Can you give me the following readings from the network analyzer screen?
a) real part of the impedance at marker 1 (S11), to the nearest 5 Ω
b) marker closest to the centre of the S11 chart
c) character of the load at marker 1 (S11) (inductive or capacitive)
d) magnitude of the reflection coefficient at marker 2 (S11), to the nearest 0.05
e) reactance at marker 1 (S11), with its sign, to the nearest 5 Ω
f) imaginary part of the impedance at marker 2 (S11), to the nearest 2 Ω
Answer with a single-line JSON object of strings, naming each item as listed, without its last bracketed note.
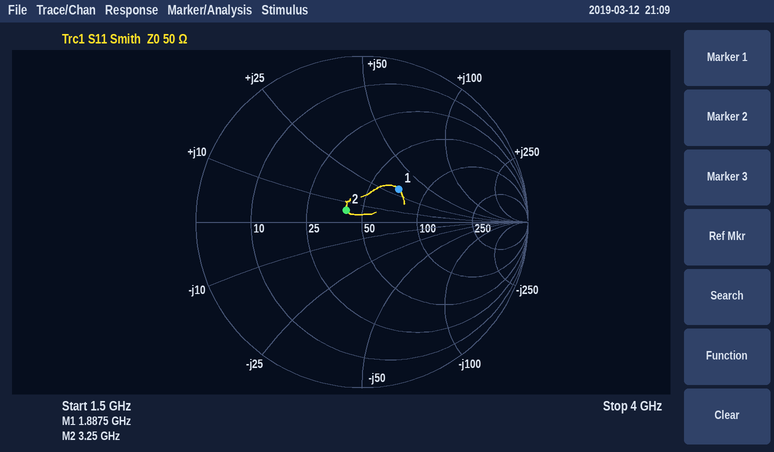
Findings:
{"real part of the impedance at marker 1 (S11), to the nearest 5 Ω": "70 Ω", "marker closest to the centre of the S11 chart": "marker 2", "character of the load at marker 1 (S11)": "inductive", "magnitude of the reflection coefficient at marker 2 (S11), to the nearest 0.05": "0.10", "reactance at marker 1 (S11), with its sign, to the nearest 5 Ω": "+30 Ω", "imaginary part of the impedance at marker 2 (S11), to the nearest 2 Ω": "+6 Ω"}
